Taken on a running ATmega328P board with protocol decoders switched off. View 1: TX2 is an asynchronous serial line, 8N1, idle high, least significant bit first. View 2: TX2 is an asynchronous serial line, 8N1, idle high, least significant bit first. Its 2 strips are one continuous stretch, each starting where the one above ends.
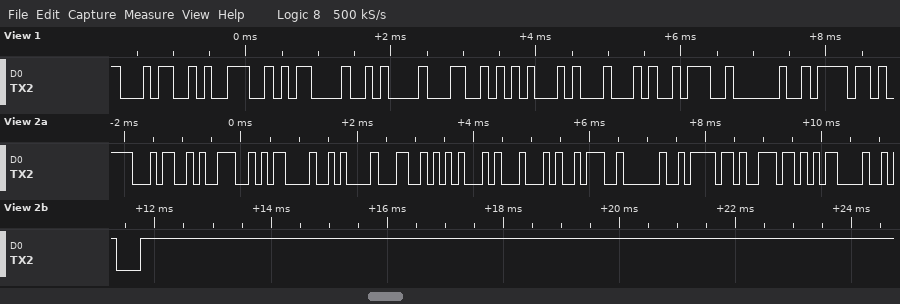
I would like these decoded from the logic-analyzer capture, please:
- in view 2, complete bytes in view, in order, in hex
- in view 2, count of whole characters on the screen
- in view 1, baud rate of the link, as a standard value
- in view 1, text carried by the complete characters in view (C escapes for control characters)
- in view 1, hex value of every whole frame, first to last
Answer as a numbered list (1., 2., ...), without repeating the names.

1. 34 39 0D 0A 4C 45 44 3A 20 6F 6E 0D 0A
2. 13
3. 9600 baud
4. "49\r\nLED: o"
5. 34 39 0D 0A 4C 45 44 3A 20 6F
